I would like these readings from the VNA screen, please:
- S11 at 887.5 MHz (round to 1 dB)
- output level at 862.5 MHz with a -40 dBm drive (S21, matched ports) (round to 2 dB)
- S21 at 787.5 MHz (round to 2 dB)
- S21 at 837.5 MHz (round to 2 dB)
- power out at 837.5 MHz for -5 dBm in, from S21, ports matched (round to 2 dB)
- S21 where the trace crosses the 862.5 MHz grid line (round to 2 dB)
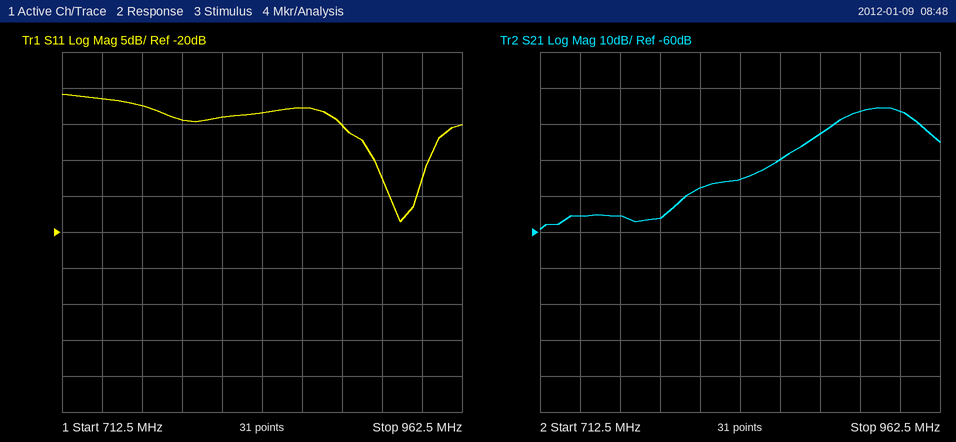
-5 dB
-80 dBm
-56 dB
-46 dB
-50 dBm
-40 dB
